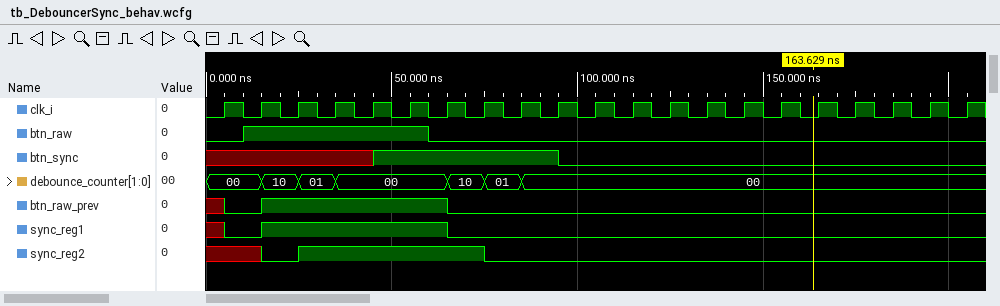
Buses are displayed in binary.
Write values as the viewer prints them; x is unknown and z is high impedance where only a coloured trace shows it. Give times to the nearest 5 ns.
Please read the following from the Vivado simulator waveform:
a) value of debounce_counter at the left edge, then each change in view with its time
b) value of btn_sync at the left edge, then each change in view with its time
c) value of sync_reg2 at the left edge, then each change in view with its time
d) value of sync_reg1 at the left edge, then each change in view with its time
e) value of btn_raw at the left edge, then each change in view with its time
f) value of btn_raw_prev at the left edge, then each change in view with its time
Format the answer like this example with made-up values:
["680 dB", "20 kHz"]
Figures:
["00, 10 at 15 ns, 01 at 25 ns, 00 at 35 ns, 10 at 65 ns, 01 at 75 ns, 00 at 85 ns", "x, 1 at 45 ns, 0 at 95 ns", "x, 0 at 15 ns, 1 at 25 ns, 0 at 75 ns", "x, 0 at 5 ns, 1 at 15 ns, 0 at 65 ns", "0, 1 at 10 ns, 0 at 60 ns", "x, 0 at 5 ns, 1 at 15 ns, 0 at 65 ns"]
